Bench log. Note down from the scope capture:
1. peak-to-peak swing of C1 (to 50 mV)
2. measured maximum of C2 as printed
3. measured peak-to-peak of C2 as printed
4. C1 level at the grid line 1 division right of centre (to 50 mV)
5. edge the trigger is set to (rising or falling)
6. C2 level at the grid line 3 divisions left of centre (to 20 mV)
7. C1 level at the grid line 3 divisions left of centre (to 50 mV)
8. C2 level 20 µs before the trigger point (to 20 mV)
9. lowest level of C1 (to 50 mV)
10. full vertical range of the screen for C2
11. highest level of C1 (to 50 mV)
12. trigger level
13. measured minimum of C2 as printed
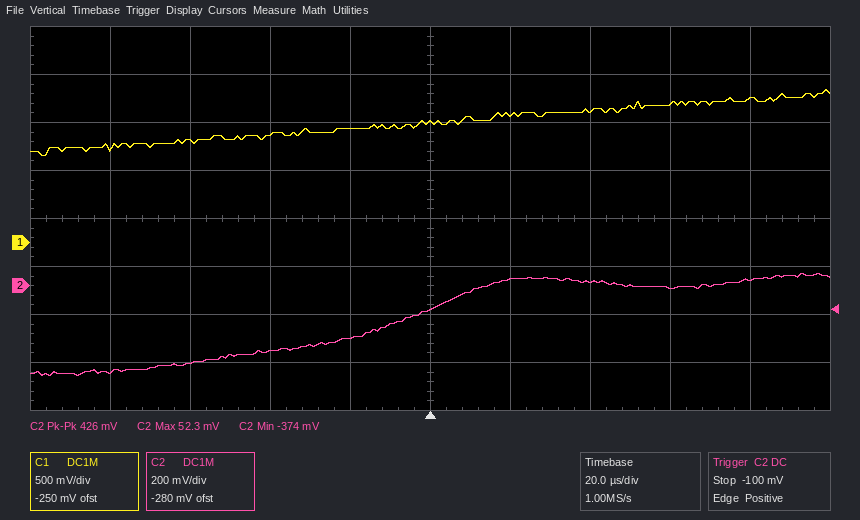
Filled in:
700 mV
52.3 mV
426 mV
1.35 V
rising
-320 mV
1.05 V
-220 mV
900 mV
1.6 V
1.60 V
-100 mV
-374 mV
